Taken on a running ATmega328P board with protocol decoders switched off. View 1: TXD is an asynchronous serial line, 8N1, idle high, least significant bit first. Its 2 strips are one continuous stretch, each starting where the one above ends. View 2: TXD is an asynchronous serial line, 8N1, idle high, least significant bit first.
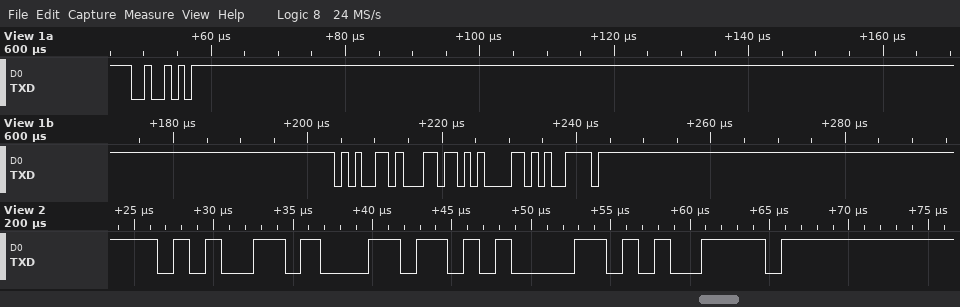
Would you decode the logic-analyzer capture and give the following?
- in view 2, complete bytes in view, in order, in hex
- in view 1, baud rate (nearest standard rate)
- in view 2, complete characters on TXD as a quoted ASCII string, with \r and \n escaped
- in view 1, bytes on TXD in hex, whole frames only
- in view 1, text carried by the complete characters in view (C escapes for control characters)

0x65 0x6C 0x61 0x79
1000000 baud
"elay"
0x52 0x65 0x6C 0x61 0x79
"Relay"
